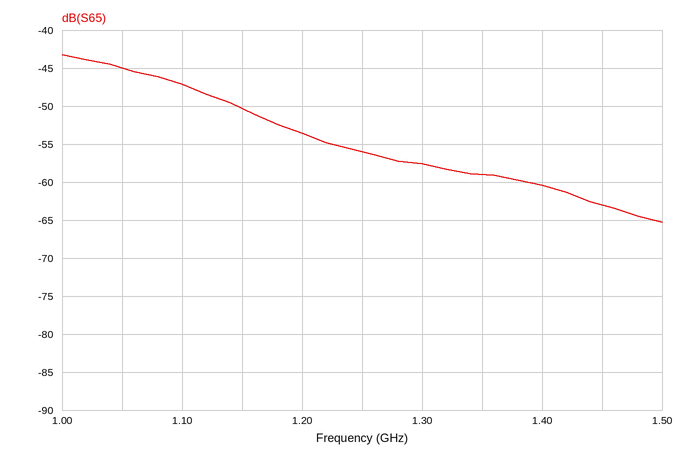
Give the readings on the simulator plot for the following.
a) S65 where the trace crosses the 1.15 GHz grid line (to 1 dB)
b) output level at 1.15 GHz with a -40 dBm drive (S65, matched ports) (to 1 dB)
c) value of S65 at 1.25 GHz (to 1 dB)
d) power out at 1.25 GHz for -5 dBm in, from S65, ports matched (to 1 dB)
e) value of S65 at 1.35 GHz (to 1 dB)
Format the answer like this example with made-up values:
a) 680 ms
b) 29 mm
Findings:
a) -50 dB
b) -90 dBm
c) -56 dB
d) -61 dBm
e) -59 dB
